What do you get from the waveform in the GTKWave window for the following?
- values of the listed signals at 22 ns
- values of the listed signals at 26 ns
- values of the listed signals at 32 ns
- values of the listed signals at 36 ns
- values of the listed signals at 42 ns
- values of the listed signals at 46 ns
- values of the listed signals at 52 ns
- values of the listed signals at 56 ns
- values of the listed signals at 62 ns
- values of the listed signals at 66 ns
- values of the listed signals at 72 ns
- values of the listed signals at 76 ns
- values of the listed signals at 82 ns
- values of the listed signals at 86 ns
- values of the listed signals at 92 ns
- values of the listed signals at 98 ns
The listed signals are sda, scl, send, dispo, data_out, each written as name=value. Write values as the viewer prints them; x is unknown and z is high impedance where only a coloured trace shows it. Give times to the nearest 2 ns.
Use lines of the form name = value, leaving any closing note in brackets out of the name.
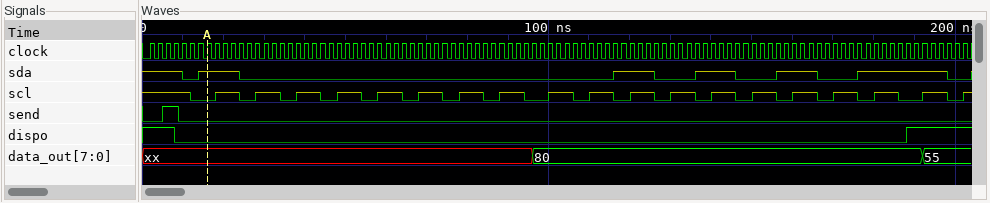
values of the listed signals at 22 ns = sda=z, scl=z, send=0, dispo=0, data_out=xx
values of the listed signals at 26 ns = sda=0, scl=0, send=0, dispo=0, data_out=xx
values of the listed signals at 32 ns = sda=0, scl=z, send=0, dispo=0, data_out=xx
values of the listed signals at 36 ns = sda=0, scl=0, send=0, dispo=0, data_out=xx
values of the listed signals at 42 ns = sda=0, scl=z, send=0, dispo=0, data_out=xx
values of the listed signals at 46 ns = sda=0, scl=0, send=0, dispo=0, data_out=xx
values of the listed signals at 52 ns = sda=0, scl=z, send=0, dispo=0, data_out=xx
values of the listed signals at 56 ns = sda=0, scl=0, send=0, dispo=0, data_out=xx
values of the listed signals at 62 ns = sda=0, scl=z, send=0, dispo=0, data_out=xx
values of the listed signals at 66 ns = sda=0, scl=0, send=0, dispo=0, data_out=xx
values of the listed signals at 72 ns = sda=0, scl=z, send=0, dispo=0, data_out=xx
values of the listed signals at 76 ns = sda=0, scl=0, send=0, dispo=0, data_out=xx
values of the listed signals at 82 ns = sda=0, scl=z, send=0, dispo=0, data_out=xx
values of the listed signals at 86 ns = sda=0, scl=0, send=0, dispo=0, data_out=xx
values of the listed signals at 92 ns = sda=0, scl=z, send=0, dispo=0, data_out=xx
values of the listed signals at 98 ns = sda=0, scl=0, send=0, dispo=0, data_out=80
